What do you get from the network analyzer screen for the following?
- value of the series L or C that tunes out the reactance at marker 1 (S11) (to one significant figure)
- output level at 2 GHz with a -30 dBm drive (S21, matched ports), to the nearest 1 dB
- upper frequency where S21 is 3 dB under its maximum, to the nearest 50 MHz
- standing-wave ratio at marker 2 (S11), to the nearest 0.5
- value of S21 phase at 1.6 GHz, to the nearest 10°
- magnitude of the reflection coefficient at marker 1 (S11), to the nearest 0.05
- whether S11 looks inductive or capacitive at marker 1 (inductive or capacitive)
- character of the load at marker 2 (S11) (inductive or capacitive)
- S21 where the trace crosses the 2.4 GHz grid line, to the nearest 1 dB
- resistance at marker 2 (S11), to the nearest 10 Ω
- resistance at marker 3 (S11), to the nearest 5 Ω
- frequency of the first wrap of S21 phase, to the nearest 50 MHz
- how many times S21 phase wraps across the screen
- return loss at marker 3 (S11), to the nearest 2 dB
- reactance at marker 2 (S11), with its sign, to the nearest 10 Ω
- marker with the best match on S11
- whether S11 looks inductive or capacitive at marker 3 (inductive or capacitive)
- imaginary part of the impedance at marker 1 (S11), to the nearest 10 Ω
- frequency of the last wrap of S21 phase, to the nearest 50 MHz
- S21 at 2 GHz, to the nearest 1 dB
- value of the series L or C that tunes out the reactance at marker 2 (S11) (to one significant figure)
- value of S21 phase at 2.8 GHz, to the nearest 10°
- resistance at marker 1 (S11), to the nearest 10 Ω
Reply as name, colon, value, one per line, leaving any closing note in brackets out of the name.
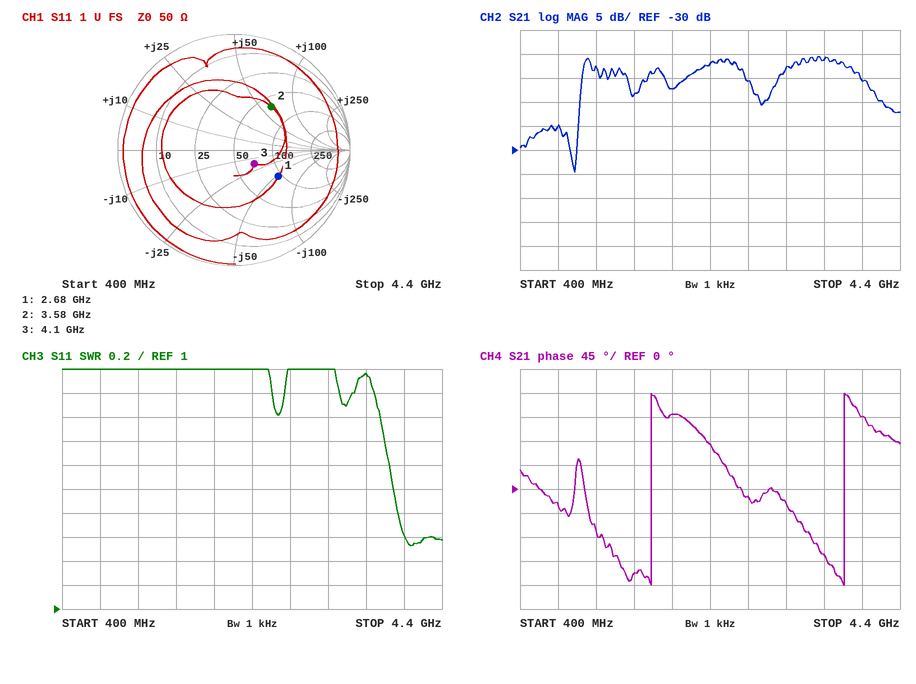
value of the series L or C that tunes out the reactance at marker 1 (S11): 3 nH
output level at 2 GHz with a -30 dBm drive (S21, matched ports), to the nearest 1 dB: -47 dBm
upper frequency where S21 is 3 dB under its maximum, to the nearest 50 MHz: 3.90 GHz
standing-wave ratio at marker 2 (S11), to the nearest 0.5: 3.0
value of S21 phase at 1.6 GHz, to the nearest 10°: -160°
magnitude of the reflection coefficient at marker 1 (S11), to the nearest 0.05: 0.45
whether S11 looks inductive or capacitive at marker 1: capacitive
character of the load at marker 2 (S11): inductive
S21 where the trace crosses the 2.4 GHz grid line, to the nearest 1 dB: -12 dB
resistance at marker 2 (S11), to the nearest 10 Ω: 60 Ω
resistance at marker 3 (S11), to the nearest 5 Ω: 70 Ω
frequency of the first wrap of S21 phase, to the nearest 50 MHz: 1.80 GHz
how many times S21 phase wraps across the screen: 2
return loss at marker 3 (S11), to the nearest 2 dB: 14 dB
reactance at marker 2 (S11), with its sign, to the nearest 10 Ω: +60 Ω
marker with the best match on S11: marker 3
whether S11 looks inductive or capacitive at marker 3: capacitive
imaginary part of the impedance at marker 1 (S11), to the nearest 10 Ω: -50 Ω
frequency of the last wrap of S21 phase, to the nearest 50 MHz: 3.80 GHz
S21 at 2 GHz, to the nearest 1 dB: -17 dB
value of the series L or C that tunes out the reactance at marker 2 (S11): 700 fF
value of S21 phase at 2.8 GHz, to the nearest 10°: -10°
resistance at marker 1 (S11), to the nearest 10 Ω: 90 Ω
